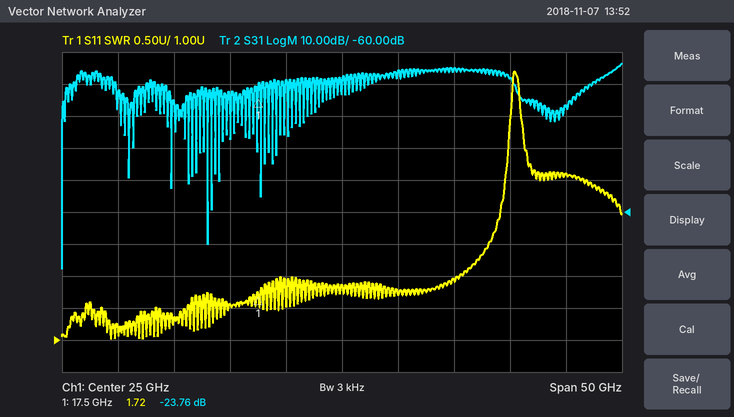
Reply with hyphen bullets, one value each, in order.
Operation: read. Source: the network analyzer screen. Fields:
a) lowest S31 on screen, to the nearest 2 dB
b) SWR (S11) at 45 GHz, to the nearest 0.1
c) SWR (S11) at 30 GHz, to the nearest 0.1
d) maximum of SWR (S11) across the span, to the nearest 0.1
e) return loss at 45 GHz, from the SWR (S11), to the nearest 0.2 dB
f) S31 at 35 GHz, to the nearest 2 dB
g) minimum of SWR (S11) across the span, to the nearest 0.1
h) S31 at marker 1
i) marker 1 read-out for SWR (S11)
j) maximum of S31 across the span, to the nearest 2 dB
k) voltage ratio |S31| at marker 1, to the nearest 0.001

- -78 dB
- 3.6
- 1.7
- 5.2
- 5.0 dB
- -16 dB
- 1.0
- -23.76 dB
- 1.72
- -14 dB
- 0.065
